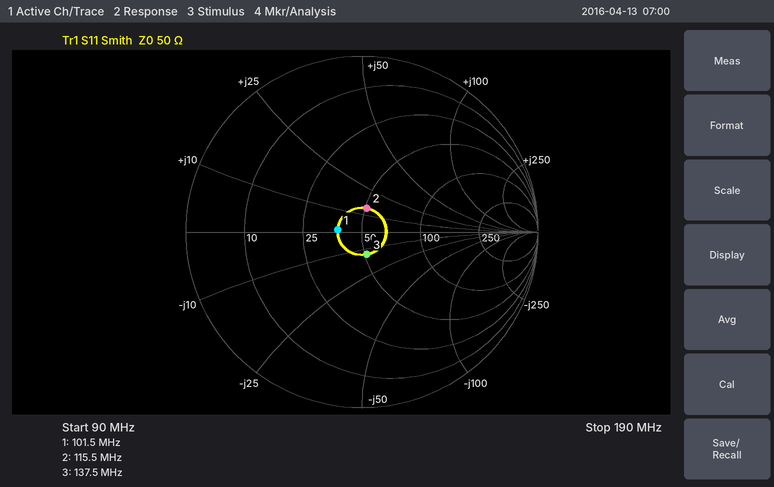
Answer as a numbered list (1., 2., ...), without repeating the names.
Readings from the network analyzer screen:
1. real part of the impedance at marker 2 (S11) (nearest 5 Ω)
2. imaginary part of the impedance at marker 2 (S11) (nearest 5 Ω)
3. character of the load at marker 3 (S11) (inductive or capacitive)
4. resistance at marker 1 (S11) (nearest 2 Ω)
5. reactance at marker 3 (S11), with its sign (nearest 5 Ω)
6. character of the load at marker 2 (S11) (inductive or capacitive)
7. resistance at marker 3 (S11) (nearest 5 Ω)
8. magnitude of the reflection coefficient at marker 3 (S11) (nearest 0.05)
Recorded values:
1. 50 Ω
2. +15 Ω
3. capacitive
4. 38 Ω
5. -15 Ω
6. inductive
7. 50 Ω
8. 0.15
